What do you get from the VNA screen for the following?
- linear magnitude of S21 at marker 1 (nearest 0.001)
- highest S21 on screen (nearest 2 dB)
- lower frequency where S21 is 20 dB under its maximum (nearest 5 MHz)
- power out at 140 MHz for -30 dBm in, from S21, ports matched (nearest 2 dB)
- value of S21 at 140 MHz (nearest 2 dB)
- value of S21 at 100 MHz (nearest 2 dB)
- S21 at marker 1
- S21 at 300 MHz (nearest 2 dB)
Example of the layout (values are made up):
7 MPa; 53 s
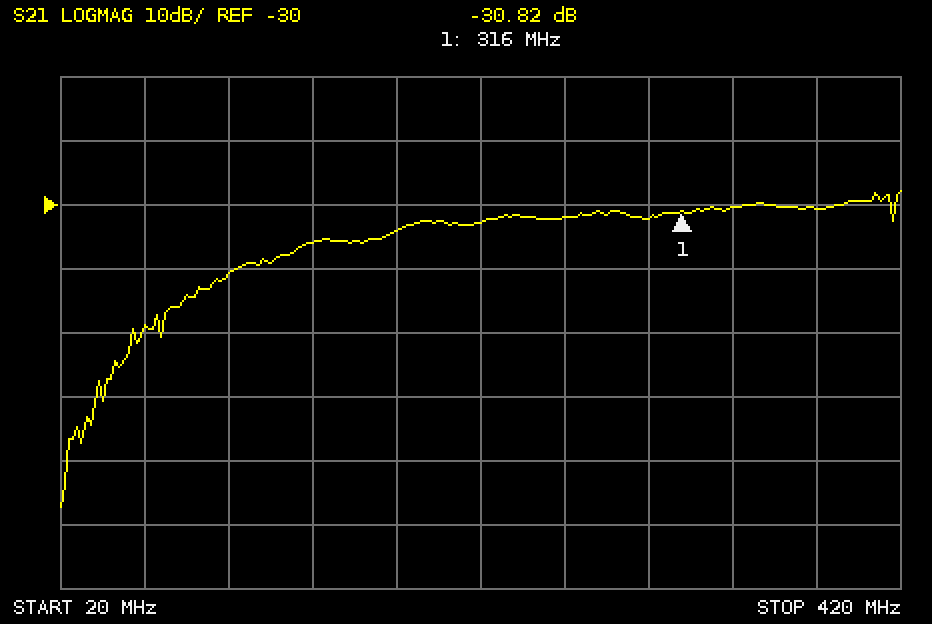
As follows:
0.029; -28 dB; 70 MHz; -66 dBm; -36 dB; -40 dB; -30.82 dB; -32 dB
